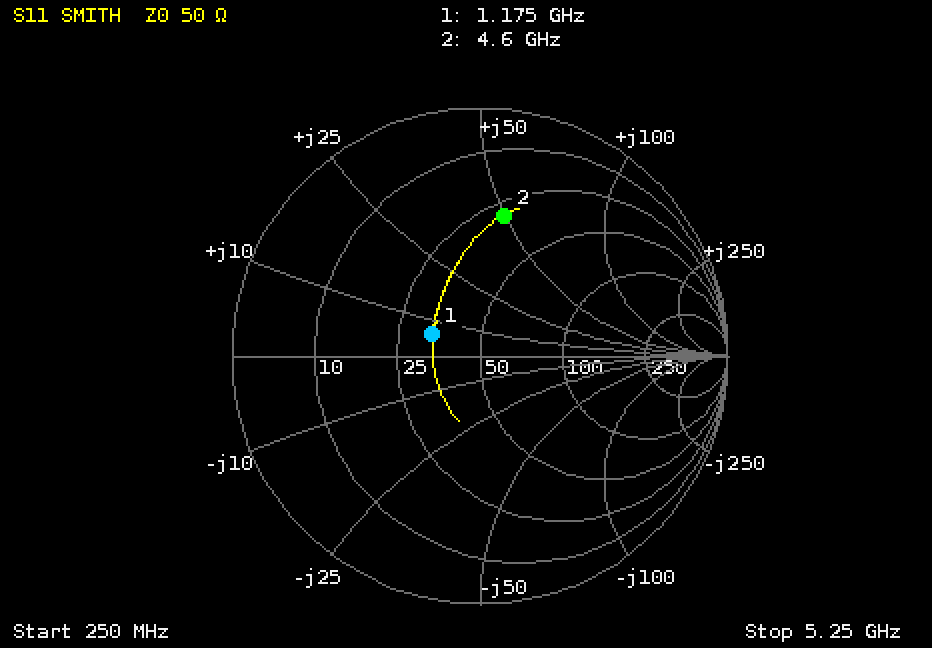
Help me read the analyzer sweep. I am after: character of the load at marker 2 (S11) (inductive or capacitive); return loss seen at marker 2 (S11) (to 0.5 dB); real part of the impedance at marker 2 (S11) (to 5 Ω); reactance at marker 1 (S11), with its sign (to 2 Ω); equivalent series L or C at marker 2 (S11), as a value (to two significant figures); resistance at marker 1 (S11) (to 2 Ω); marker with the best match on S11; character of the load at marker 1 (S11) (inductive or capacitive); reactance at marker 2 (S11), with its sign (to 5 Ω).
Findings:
inductive
5.0 dB
30 Ω
+6 Ω
1.7 nH
34 Ω
marker 1
inductive
+50 Ω
